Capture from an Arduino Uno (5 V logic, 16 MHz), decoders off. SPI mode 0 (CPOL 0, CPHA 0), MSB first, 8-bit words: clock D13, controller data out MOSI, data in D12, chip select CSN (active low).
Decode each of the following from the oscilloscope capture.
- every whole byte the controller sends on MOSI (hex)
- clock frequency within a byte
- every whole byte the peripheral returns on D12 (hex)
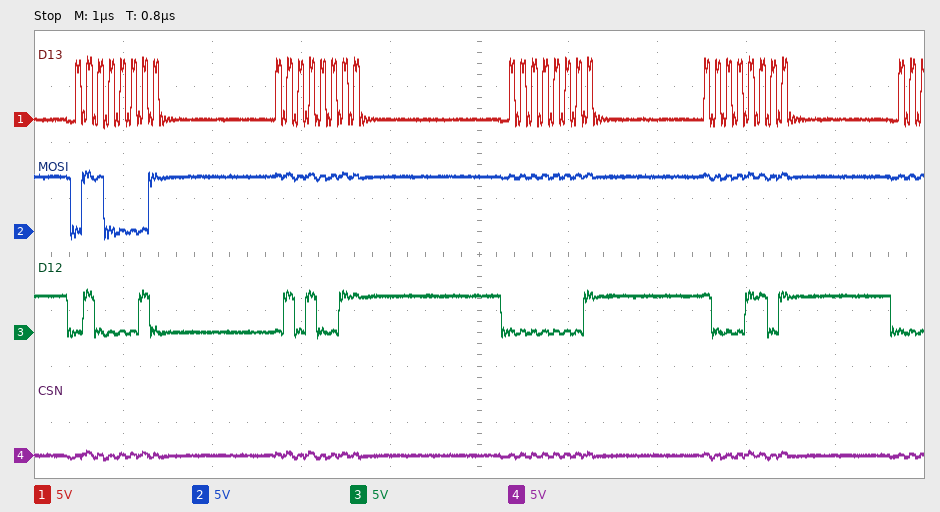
61 FF FF FF
8 MHz
42 53 01 8D
